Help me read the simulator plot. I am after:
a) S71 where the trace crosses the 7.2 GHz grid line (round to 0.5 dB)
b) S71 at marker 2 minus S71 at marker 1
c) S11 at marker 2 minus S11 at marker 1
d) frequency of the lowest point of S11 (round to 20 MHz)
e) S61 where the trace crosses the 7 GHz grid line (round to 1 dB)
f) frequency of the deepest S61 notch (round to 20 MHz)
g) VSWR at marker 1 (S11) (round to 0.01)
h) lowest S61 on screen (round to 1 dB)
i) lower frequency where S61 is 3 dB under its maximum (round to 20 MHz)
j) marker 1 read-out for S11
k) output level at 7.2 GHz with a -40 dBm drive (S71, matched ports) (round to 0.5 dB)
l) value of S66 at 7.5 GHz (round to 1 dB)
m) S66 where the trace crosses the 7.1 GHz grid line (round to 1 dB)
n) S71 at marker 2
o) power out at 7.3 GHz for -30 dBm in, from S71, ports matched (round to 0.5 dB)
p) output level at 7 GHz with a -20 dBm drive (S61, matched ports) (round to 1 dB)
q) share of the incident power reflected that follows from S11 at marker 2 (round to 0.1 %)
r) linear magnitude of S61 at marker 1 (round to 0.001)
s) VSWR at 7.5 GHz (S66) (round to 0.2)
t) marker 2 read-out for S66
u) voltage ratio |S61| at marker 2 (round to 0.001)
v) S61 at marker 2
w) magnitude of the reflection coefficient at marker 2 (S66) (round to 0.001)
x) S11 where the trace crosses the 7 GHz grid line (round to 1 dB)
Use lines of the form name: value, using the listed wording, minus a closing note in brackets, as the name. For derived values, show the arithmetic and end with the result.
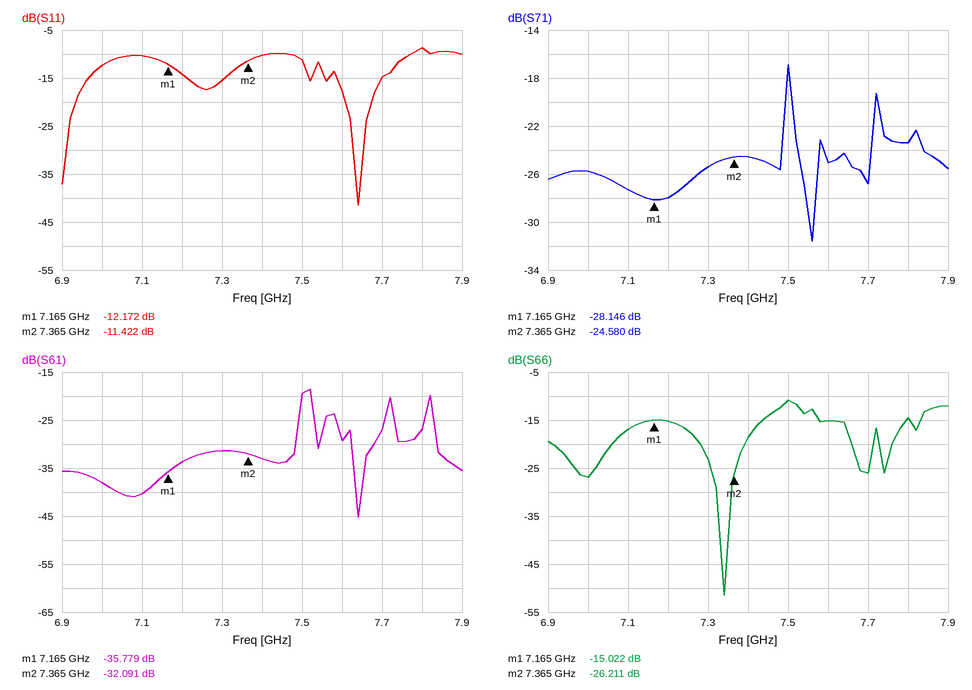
S71 where the trace crosses the 7.2 GHz grid line: -28.0 dB
S71 at marker 2 minus S71 at marker 1: -24.58 − (-28.146) = 3.566 dB
S11 at marker 2 minus S11 at marker 1: -11.422 − (-12.172) = 0.750 dB
frequency of the lowest point of S11: 7.64 GHz
S61 where the trace crosses the 7 GHz grid line: -38 dB
frequency of the deepest S61 notch: 7.64 GHz
VSWR at marker 1 (S11): (1 + 0.2463)/(1 − 0.2463) ≈ 1.65
lowest S61 on screen: -45 dB
lower frequency where S61 is 3 dB under its maximum: 7.50 GHz
marker 1 read-out for S11: -12.172 dB
output level at 7.2 GHz with a -40 dBm drive (S71, matched ports): -40 dBm + (-28.0 dB) = -68.0 dBm
value of S66 at 7.5 GHz: -11 dB
S66 where the trace crosses the 7.1 GHz grid line: -17 dB
S71 at marker 2: -24.580 dB
power out at 7.3 GHz for -30 dBm in, from S71, ports matched: -30 dBm + (-25.5 dB) = -55.5 dBm
output level at 7 GHz with a -20 dBm drive (S61, matched ports): -20 dBm + (-38 dB) = -58 dBm
share of the incident power reflected that follows from S11 at marker 2: 10^(-11.422/10) ≈ 7.2 %
linear magnitude of S61 at marker 1: 10^(-35.779/20) ≈ 0.016
VSWR at 7.5 GHz (S66): |Γ| = 10^(-11/20) = 0.2818; VSWR = (1 + 0.2818)/(1 − 0.2818) ≈ 1.8
marker 2 read-out for S66: -26.211 dB
voltage ratio |S61| at marker 2: 10^(-32.091/20) ≈ 0.025
S61 at marker 2: -32.091 dB
magnitude of the reflection coefficient at marker 2 (S66): 10^(-26.211/20) ≈ 0.049
S11 where the trace crosses the 7 GHz grid line: -12 dB
